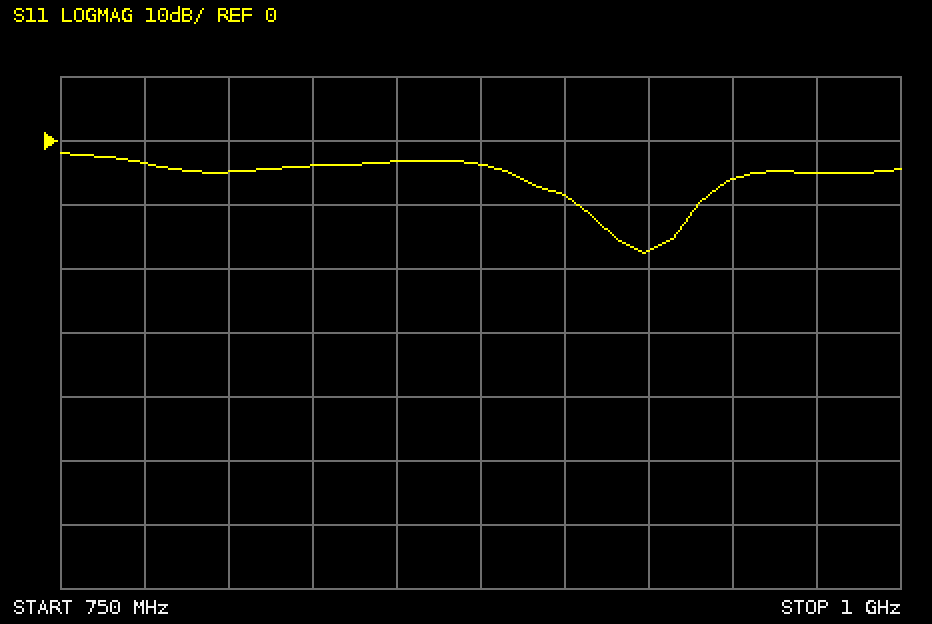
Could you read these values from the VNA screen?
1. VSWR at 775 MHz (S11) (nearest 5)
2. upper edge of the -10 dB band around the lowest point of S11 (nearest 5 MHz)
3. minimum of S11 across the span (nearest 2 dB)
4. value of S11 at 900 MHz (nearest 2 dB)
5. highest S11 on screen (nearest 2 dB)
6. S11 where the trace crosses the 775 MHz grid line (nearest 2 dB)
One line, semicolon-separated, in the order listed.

5; 940 MHz; -18 dB; -8 dB; -2 dB; -4 dB
